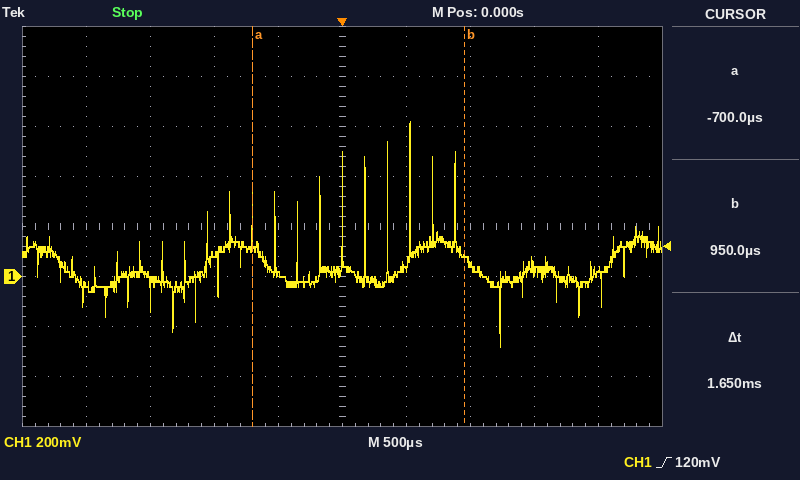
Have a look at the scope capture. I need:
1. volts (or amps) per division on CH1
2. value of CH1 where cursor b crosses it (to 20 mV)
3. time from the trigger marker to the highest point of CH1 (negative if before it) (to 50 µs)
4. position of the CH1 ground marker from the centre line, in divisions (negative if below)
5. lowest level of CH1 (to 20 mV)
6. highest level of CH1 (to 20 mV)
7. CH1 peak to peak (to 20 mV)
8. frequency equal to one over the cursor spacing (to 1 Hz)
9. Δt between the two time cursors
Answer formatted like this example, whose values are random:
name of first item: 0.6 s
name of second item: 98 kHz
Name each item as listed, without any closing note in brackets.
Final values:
volts (or amps) per division on CH1: 200 mV
value of CH1 where cursor b crosses it: 80 mV
time from the trigger marker to the highest point of CH1 (negative if before it): +550 µs
position of the CH1 ground marker from the centre line, in divisions: -1.0 div
lowest level of CH1: -280 mV
highest level of CH1: 620 mV
CH1 peak to peak: 900 mV
frequency equal to one over the cursor spacing: 606 Hz
Δt between the two time cursors: 1.65 ms
